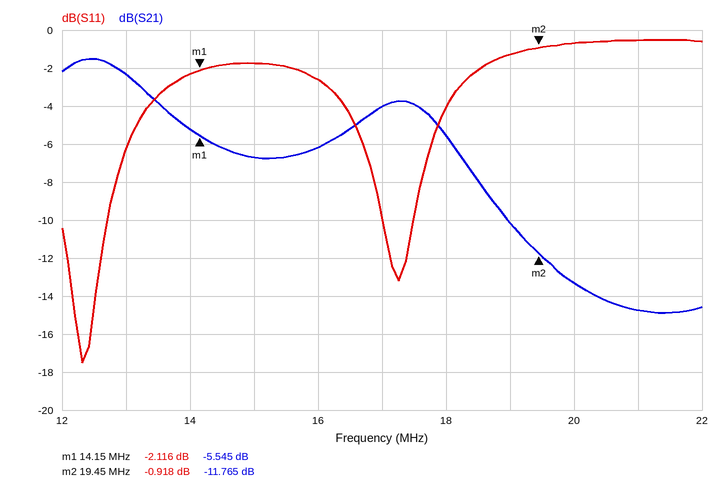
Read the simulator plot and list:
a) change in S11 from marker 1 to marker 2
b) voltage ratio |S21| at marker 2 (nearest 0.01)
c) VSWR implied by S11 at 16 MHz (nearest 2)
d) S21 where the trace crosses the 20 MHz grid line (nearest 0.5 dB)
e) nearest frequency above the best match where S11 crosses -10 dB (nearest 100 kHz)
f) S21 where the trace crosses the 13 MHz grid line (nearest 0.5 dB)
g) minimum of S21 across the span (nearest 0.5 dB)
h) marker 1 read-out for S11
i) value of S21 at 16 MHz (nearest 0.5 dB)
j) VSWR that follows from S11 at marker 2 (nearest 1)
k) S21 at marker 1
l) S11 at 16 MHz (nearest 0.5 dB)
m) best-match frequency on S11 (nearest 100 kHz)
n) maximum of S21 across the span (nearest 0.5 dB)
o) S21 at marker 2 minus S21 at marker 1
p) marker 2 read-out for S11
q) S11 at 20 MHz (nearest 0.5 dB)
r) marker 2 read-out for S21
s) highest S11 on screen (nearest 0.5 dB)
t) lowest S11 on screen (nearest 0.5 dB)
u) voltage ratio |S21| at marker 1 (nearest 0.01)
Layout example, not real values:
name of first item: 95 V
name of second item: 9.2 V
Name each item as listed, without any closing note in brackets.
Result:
change in S11 from marker 1 to marker 2: 1.198 dB
voltage ratio |S21| at marker 2: 0.26
VSWR implied by S11 at 16 MHz: 6
S21 where the trace crosses the 20 MHz grid line: -13.5 dB
nearest frequency above the best match where S11 crosses -10 dB: 12.7 MHz
S21 where the trace crosses the 13 MHz grid line: -2.5 dB
minimum of S21 across the span: -15.0 dB
marker 1 read-out for S11: -2.116 dB
value of S21 at 16 MHz: -6.0 dB
VSWR that follows from S11 at marker 2: 19
S21 at marker 1: -5.545 dB
S11 at 16 MHz: -2.5 dB
best-match frequency on S11: 12.3 MHz
maximum of S21 across the span: -1.5 dB
S21 at marker 2 minus S21 at marker 1: -6.220 dB
marker 2 read-out for S11: -0.918 dB
S11 at 20 MHz: -0.5 dB
marker 2 read-out for S21: -11.765 dB
highest S11 on screen: -0.5 dB
lowest S11 on screen: -17.5 dB
voltage ratio |S21| at marker 1: 0.53
